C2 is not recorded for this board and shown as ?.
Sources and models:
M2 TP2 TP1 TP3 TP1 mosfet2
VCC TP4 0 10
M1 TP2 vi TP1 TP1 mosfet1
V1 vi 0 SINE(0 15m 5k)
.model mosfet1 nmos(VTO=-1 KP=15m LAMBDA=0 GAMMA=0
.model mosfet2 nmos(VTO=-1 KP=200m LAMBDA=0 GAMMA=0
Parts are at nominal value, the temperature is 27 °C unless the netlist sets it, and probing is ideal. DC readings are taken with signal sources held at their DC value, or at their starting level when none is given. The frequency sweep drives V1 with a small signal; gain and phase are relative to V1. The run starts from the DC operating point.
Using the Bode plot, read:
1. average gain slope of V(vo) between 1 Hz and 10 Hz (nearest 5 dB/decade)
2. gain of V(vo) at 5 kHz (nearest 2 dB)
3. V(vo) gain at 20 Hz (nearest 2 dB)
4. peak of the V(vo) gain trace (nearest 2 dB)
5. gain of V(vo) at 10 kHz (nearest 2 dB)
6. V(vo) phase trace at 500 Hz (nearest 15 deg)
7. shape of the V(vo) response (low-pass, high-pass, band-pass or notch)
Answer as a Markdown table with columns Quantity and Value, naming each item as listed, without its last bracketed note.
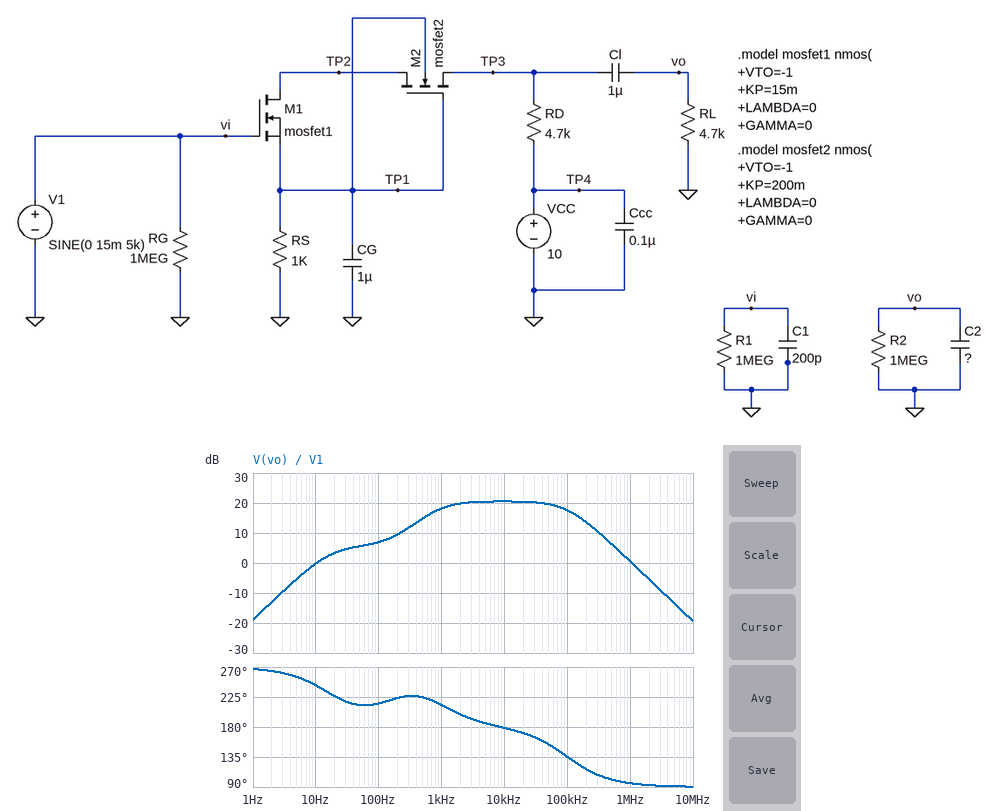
| Quantity | Value |
|---|---|
| average gain slope of V(vo) between 1 Hz and 10 Hz | 20 dB/decade |
| gain of V(vo) at 5 kHz | 20 dB |
| V(vo) gain at 20 Hz | 4 dB |
| peak of the V(vo) gain trace | 20 dB |
| gain of V(vo) at 10 kHz | 20 dB |
| V(vo) phase trace at 500 Hz | 225 deg |
| shape of the V(vo) response | band-pass |
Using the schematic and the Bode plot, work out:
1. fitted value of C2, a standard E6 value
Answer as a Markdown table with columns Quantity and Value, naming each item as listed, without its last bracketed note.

| Quantity | Value |
|---|---|
| fitted value of C2, a standard E6 value | 680 pF |
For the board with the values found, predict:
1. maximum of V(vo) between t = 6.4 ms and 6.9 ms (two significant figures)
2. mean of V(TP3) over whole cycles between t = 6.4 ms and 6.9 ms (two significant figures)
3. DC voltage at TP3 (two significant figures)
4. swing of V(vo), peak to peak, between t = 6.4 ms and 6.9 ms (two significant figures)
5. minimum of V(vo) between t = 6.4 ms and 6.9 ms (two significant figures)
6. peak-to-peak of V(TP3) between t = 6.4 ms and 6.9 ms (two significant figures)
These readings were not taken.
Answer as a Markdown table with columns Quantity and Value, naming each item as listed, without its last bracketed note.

| Quantity | Value |
|---|---|
| maximum of V(vo) between t = 6.4 ms and 6.9 ms | 160 mV |
| mean of V(TP3) over whole cycles between t = 6.4 ms and 6.9 ms | 6.7 V |
| DC voltage at TP3 | 6.7 V |
| swing of V(vo), peak to peak, between t = 6.4 ms and 6.9 ms | 320 mV |
| minimum of V(vo) between t = 6.4 ms and 6.9 ms | -160 mV |
| peak-to-peak of V(TP3) between t = 6.4 ms and 6.9 ms | 320 mV |
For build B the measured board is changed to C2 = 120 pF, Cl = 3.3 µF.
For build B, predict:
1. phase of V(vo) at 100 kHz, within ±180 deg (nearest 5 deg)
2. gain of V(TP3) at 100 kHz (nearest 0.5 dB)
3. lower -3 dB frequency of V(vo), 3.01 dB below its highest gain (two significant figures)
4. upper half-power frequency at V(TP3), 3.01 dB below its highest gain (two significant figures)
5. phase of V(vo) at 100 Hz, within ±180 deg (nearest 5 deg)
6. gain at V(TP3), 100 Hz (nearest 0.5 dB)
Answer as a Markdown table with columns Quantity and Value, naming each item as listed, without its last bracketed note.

| Quantity | Value |
|---|---|
| phase of V(vo) at 100 kHz, within ±180 deg | 170 deg |
| gain of V(TP3) at 100 kHz | 20.5 dB |
| lower -3 dB frequency of V(vo), 3.01 dB below its highest gain | 850 Hz |
| upper half-power frequency at V(TP3), 3.01 dB below its highest gain | 570 kHz |
| phase of V(vo) at 100 Hz, within ±180 deg | -150 deg |
| gain at V(TP3), 100 Hz | 7.0 dB |
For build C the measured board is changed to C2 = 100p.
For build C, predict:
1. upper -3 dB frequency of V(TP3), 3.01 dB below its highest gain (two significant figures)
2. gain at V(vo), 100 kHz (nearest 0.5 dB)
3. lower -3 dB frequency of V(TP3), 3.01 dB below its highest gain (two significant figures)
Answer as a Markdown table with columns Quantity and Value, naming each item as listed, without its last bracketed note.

| Quantity | Value |
|---|---|
| upper -3 dB frequency of V(TP3), 3.01 dB below its highest gain | 680 kHz |
| gain at V(vo), 100 kHz | 20.5 dB |
| lower -3 dB frequency of V(TP3), 3.01 dB below its highest gain | 850 Hz |
